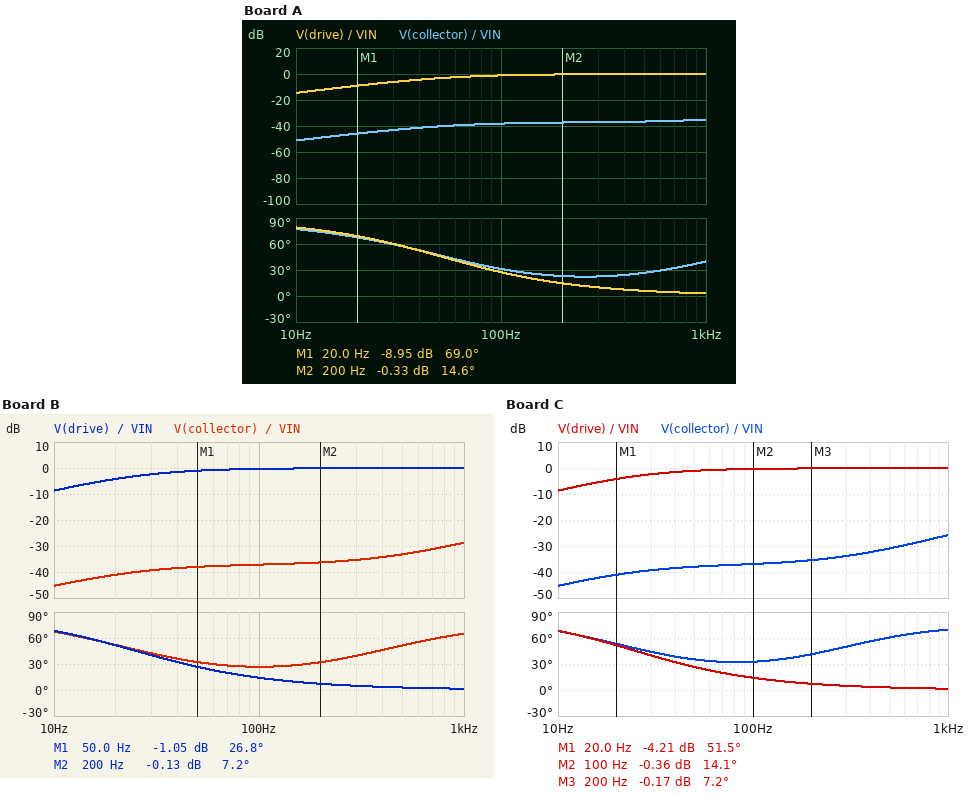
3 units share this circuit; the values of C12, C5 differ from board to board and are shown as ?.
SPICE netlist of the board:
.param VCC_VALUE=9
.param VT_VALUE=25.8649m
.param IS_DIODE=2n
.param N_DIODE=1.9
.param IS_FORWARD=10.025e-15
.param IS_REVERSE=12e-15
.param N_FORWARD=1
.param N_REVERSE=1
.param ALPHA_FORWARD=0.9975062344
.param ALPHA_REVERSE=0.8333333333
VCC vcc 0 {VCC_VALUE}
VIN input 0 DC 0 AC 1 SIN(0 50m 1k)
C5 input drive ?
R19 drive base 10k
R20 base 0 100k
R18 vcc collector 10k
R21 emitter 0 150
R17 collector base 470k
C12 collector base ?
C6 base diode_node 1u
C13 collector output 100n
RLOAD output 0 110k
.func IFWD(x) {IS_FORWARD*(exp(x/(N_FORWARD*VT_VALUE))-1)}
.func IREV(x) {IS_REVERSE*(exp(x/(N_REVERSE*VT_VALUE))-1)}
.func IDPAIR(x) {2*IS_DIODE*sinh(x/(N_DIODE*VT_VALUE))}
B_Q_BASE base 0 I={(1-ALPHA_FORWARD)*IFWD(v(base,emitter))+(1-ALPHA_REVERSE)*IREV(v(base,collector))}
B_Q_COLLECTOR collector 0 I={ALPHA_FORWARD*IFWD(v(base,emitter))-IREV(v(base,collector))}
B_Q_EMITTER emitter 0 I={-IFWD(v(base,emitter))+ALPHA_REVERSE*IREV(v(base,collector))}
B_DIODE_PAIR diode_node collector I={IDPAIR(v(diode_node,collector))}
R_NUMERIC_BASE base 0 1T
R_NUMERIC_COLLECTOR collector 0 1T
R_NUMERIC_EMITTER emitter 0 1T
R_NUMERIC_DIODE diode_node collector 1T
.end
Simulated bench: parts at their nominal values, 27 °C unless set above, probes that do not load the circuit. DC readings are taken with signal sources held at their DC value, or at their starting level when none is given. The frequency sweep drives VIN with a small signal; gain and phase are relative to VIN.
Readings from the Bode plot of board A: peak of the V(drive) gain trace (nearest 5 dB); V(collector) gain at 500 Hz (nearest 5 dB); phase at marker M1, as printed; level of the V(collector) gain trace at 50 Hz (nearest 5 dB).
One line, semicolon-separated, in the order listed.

0 dB; -35 dB; 69.0 deg; -40 dB
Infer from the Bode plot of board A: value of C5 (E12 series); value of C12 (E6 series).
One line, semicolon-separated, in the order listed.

33 nF; 220 pF
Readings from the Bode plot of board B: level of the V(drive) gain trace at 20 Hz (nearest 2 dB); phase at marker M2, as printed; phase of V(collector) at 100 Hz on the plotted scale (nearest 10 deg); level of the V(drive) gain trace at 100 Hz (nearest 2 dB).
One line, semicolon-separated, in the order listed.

-4 dB; 7.2 deg; 30 deg; 0 dB
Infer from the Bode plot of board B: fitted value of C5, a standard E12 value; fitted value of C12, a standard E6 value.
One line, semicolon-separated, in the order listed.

68 nF; 680 pF
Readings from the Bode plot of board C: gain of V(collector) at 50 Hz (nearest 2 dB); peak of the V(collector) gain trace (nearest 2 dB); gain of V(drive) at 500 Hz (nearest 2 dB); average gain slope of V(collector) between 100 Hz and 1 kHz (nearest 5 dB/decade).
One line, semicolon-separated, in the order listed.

-38 dB; -26 dB; 0 dB; 10 dB/decade
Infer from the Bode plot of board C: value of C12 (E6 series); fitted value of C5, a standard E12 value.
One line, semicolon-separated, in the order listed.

1 nF; 68 nF
